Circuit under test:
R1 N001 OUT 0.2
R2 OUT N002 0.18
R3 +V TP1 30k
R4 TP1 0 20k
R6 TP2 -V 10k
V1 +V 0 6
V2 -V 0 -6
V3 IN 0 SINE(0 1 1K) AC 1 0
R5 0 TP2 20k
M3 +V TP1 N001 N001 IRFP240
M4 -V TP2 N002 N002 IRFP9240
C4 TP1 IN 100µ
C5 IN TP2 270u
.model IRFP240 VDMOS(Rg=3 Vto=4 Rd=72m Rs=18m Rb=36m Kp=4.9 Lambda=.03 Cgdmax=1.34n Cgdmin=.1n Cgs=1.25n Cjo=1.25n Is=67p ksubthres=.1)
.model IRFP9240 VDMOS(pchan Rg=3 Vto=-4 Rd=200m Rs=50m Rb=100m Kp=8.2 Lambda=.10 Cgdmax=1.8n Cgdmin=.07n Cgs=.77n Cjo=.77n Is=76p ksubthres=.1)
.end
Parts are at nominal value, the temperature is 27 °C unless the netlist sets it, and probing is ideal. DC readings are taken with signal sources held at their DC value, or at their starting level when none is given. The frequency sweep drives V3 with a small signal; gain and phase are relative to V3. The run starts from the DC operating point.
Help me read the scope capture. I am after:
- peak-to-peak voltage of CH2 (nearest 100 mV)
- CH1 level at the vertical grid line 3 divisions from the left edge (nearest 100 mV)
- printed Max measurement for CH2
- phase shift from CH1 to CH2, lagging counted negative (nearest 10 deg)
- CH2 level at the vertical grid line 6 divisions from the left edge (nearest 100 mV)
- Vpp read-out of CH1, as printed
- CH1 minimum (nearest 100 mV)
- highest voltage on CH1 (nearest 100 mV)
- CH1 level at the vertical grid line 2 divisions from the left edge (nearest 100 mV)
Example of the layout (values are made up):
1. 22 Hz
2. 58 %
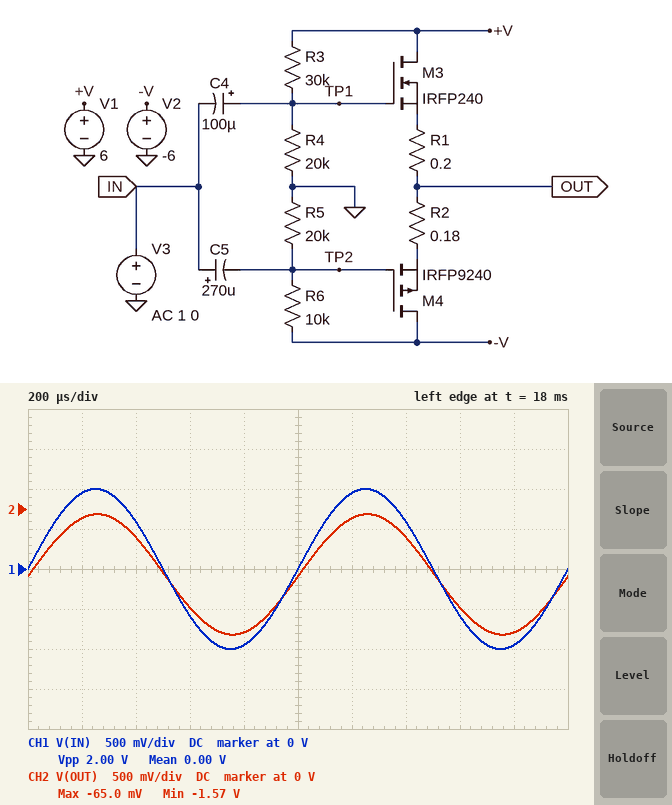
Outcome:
1. 1.5 V
2. -600 mV
3. -65.0 mV
4. 0 deg
5. -100 mV
6. 2.00 V
7. -1.0 V
8. 1.0 V
9. 600 mV
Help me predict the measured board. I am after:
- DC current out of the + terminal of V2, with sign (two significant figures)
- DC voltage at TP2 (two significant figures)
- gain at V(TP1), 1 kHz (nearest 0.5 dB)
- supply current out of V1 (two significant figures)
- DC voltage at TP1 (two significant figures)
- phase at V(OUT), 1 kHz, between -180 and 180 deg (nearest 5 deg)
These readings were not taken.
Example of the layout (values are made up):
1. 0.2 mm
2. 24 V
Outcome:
1. -200 µA
2. -4.0 V
3. 0 dB
4. 120 µA
5. 2.4 V
6. 0 deg
